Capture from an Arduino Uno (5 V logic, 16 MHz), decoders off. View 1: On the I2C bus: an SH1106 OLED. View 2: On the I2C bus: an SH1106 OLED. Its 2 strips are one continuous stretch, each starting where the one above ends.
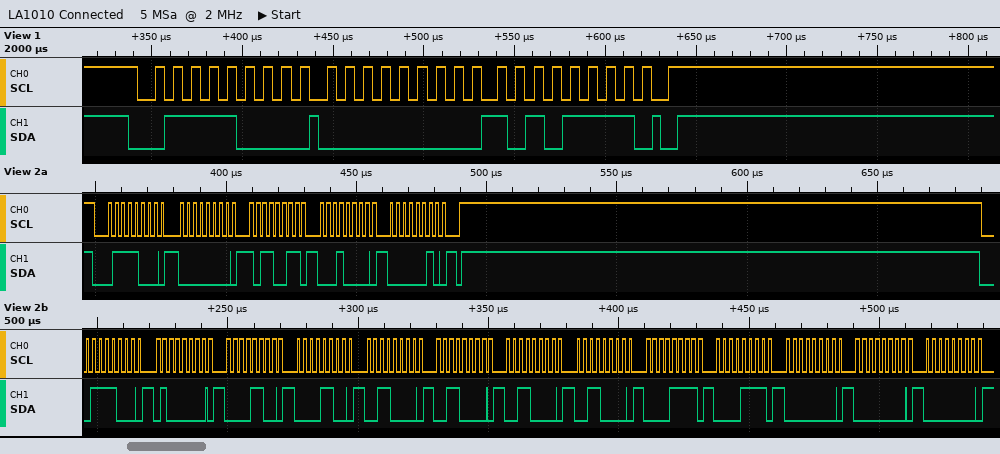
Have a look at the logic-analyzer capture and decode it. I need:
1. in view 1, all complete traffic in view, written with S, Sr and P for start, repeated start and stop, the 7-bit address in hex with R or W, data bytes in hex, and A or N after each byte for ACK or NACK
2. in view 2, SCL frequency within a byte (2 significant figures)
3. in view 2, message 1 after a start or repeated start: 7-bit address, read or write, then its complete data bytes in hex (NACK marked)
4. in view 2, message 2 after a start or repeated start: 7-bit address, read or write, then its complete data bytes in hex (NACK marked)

S 3CW A 00 A AF A P
400 kHz
0x3C write: 00 B3 10 02
0x3C write: 40 0C 0C 30 30 30 30 0F 0F 00 00 00
